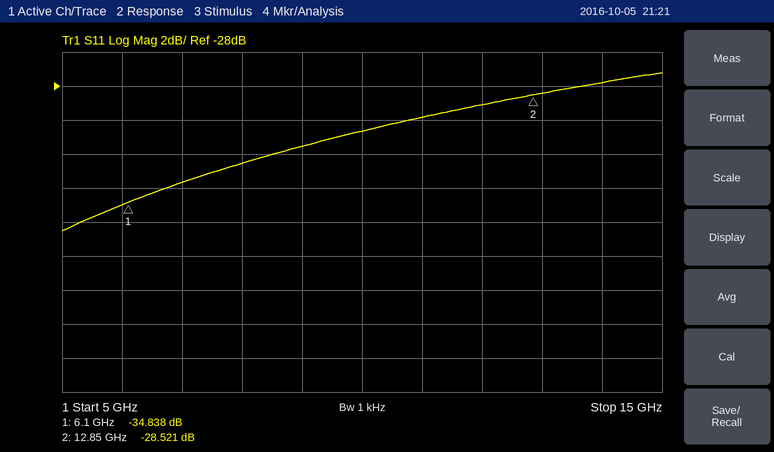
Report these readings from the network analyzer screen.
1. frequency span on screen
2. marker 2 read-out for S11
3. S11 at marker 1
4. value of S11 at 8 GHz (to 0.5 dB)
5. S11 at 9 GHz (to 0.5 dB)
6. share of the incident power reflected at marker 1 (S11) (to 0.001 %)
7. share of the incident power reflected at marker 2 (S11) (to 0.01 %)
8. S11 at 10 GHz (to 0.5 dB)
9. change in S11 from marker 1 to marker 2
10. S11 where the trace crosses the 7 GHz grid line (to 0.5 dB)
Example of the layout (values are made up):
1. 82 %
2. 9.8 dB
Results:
1. 10 GHz
2. -28.521 dB
3. -34.838 dB
4. -32.5 dB
5. -31.5 dB
6. 0.033 %
7. 0.14 %
8. -30.5 dB
9. 6.317 dB
10. -33.5 dB
